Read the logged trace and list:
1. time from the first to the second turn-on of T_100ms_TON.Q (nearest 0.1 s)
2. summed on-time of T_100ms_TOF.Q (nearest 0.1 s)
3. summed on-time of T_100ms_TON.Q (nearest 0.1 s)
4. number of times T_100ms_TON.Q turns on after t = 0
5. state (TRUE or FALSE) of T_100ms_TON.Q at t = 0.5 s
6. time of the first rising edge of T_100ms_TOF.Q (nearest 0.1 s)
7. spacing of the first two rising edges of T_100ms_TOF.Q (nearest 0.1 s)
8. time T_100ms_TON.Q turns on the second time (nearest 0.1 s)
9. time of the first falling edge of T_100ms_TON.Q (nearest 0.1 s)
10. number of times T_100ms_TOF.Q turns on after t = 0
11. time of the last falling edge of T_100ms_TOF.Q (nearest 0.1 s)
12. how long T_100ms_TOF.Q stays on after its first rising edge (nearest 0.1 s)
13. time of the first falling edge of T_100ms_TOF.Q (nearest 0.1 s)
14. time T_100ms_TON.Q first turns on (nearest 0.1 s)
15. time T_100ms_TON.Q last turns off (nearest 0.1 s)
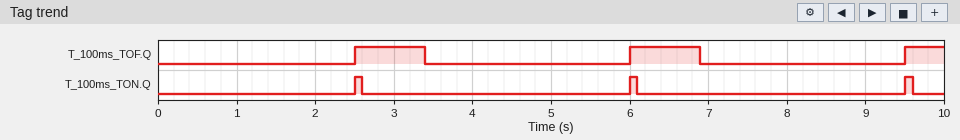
3.5 s
2.3 s
0.3 s
3
FALSE
2.5 s
3.5 s
6.0 s
2.6 s
3
6.9 s
0.9 s
3.4 s
2.5 s
9.6 s
